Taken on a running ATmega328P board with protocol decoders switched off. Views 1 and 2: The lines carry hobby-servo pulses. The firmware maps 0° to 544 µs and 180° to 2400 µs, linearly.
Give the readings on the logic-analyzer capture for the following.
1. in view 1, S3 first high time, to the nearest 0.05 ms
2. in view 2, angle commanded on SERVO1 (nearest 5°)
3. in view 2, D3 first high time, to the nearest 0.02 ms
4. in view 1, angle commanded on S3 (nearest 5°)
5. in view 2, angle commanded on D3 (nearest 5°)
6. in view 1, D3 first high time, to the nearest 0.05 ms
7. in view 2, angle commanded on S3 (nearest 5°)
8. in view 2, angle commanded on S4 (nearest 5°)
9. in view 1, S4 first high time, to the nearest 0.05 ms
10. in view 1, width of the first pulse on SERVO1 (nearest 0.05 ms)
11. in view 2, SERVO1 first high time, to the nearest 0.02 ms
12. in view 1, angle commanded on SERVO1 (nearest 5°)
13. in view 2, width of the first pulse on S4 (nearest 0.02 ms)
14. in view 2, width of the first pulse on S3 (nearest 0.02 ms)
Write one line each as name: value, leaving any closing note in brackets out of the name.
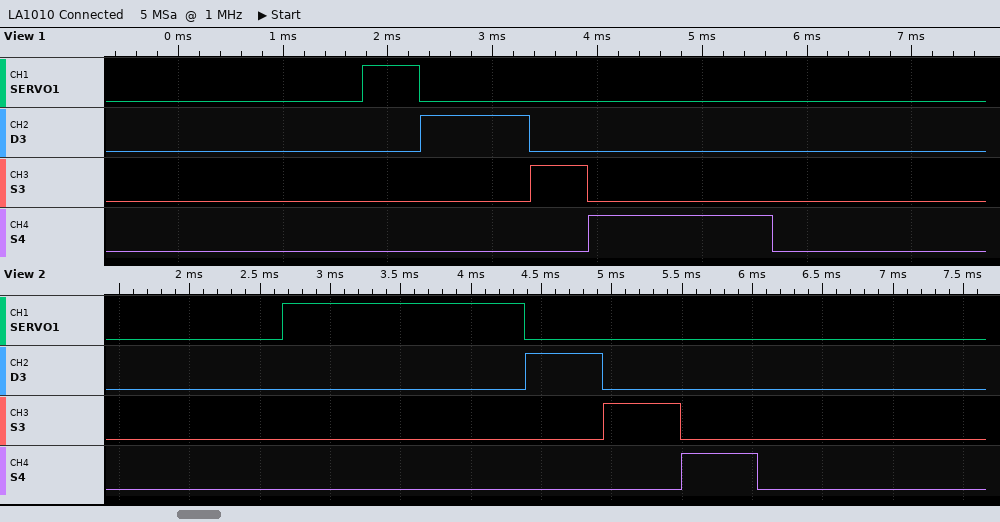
in view 1, S3 first high time, to the nearest 0.05 ms: 0.55 ms
in view 2, angle commanded on SERVO1: 115°
in view 2, D3 first high time, to the nearest 0.02 ms: 0.54 ms
in view 1, angle commanded on S3: 0°
in view 2, angle commanded on D3: 0°
in view 1, D3 first high time, to the nearest 0.05 ms: 1.05 ms
in view 2, angle commanded on S3: 0°
in view 2, angle commanded on S4: 0°
in view 1, S4 first high time, to the nearest 0.05 ms: 1.75 ms
in view 1, width of the first pulse on SERVO1: 0.55 ms
in view 2, SERVO1 first high time, to the nearest 0.02 ms: 1.72 ms
in view 1, angle commanded on SERVO1: 0°
in view 2, width of the first pulse on S4: 0.54 ms
in view 2, width of the first pulse on S3: 0.54 ms
